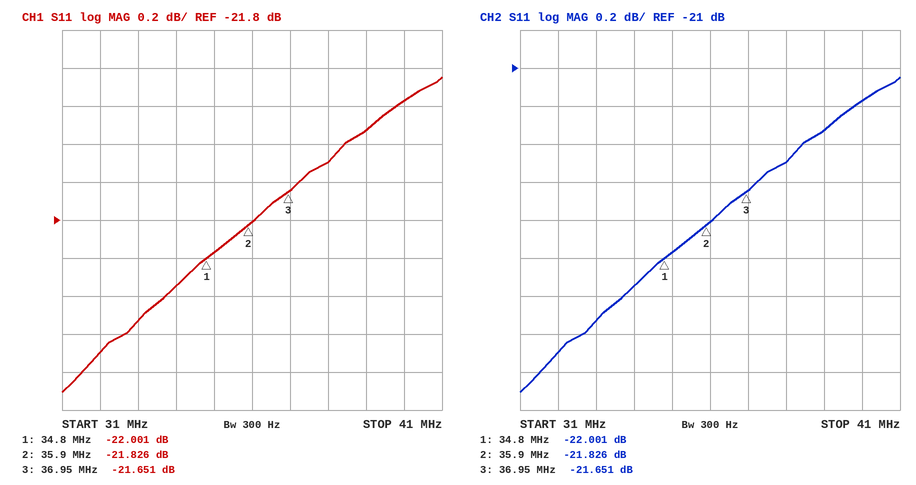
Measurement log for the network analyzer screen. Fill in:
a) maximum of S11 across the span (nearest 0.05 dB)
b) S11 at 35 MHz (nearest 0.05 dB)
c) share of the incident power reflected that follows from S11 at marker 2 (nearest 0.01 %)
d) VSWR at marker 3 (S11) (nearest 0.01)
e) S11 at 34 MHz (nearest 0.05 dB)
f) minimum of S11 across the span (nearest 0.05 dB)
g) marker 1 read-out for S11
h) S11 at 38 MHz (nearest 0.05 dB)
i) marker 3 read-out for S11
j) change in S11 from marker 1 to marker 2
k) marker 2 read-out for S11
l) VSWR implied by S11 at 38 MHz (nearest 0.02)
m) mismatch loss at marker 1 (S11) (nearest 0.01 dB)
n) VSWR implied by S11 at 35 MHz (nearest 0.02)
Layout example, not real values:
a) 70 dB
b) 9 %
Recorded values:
a) -21.05 dB
b) -21.95 dB
c) 0.66 %
d) 1.18
e) -22.15 dB
f) -22.70 dB
g) -22.001 dB
h) -21.50 dB
i) -21.651 dB
j) 0.175 dB
k) -21.826 dB
l) 1.18
m) 0.03 dB
n) 1.18
